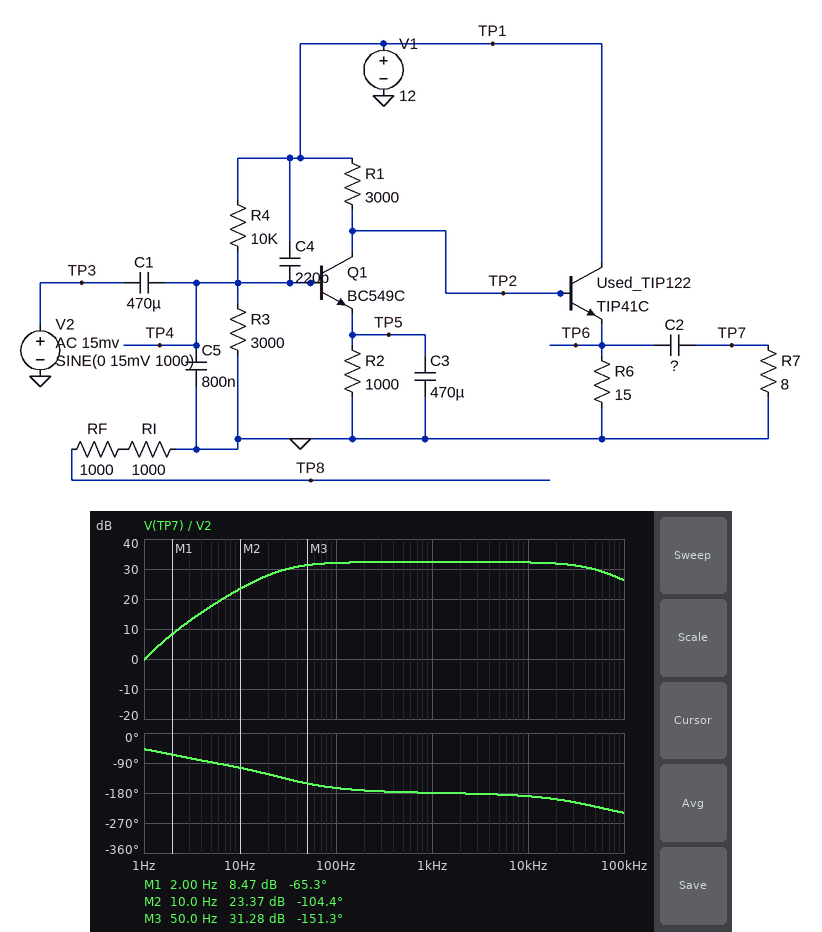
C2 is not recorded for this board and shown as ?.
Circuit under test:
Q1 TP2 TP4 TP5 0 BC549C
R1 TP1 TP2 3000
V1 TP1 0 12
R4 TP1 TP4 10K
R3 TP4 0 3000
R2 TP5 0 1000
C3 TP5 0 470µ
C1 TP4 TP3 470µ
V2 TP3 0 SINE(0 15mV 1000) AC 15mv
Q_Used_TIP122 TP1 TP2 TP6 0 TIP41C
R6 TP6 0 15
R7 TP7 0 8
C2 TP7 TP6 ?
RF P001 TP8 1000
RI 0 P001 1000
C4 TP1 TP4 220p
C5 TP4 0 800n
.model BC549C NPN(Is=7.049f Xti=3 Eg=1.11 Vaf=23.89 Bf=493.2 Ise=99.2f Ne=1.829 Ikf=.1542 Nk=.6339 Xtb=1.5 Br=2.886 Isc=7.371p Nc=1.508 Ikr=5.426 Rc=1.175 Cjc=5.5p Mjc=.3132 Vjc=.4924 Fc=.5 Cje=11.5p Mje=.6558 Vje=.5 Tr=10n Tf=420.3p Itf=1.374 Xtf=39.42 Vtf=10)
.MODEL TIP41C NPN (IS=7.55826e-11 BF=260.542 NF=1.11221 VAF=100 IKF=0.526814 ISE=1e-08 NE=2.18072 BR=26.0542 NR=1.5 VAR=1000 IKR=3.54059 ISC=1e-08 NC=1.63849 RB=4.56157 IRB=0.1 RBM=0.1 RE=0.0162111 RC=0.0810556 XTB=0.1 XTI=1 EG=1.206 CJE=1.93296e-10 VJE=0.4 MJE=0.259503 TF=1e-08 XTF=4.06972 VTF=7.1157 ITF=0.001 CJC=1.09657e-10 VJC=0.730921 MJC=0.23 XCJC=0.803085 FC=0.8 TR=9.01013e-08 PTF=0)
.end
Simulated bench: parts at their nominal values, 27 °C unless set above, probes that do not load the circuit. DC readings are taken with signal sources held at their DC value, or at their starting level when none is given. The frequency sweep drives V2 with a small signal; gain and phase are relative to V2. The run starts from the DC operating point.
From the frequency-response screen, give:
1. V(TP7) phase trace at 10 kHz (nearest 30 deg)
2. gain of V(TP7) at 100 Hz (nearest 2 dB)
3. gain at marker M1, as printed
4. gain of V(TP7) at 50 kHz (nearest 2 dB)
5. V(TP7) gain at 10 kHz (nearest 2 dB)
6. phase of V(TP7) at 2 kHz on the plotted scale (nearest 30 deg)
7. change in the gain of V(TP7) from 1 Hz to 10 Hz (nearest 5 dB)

-180 deg
32 dB
8.47 dB
30 dB
32 dB
-180 deg
25 dB
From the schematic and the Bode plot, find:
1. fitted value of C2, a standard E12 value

6.8 mF
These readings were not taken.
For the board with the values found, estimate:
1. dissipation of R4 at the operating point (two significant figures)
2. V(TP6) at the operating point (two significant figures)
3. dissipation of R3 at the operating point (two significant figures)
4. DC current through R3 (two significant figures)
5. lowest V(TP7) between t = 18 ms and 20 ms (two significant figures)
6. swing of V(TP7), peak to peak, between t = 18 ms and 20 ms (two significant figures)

8.5 mW
1.9 V
2.5 mW
920 µA
-390 mV
880 mV
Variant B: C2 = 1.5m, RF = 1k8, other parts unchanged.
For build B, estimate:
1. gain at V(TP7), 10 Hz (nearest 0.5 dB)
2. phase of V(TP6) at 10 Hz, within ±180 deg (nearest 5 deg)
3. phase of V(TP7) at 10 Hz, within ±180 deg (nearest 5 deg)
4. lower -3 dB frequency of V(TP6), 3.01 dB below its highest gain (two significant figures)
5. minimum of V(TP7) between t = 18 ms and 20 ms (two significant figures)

22.0 dB
-135 deg
-80 deg
21 Hz
-410 mV
